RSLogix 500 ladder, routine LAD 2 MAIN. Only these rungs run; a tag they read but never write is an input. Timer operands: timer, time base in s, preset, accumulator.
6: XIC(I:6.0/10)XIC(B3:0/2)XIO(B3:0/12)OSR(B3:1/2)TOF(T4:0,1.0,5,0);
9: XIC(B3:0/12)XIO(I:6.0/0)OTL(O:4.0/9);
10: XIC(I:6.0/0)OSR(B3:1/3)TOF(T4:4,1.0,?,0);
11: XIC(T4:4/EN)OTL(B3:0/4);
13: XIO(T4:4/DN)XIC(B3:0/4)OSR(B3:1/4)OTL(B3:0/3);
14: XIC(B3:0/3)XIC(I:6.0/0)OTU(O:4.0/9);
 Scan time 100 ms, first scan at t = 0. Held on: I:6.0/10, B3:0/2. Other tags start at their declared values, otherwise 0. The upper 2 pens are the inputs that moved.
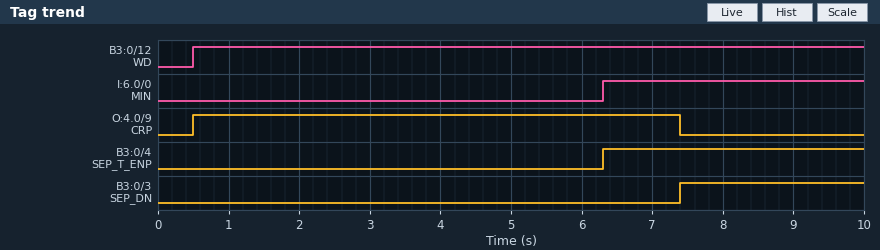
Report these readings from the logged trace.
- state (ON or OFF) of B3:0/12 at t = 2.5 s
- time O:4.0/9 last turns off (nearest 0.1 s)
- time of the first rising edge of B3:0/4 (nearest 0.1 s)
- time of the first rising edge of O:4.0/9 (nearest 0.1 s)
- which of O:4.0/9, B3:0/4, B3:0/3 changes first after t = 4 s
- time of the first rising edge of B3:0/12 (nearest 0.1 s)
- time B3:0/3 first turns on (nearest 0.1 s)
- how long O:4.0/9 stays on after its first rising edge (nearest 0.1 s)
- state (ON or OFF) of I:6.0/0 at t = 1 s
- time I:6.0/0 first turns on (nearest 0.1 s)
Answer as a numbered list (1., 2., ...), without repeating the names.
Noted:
1. ON
2. 7.4 s
3. 6.3 s
4. 0.5 s
5. B3:0/4
6. 0.5 s
7. 7.4 s
8. 6.9 s
9. OFF
10. 6.3 s
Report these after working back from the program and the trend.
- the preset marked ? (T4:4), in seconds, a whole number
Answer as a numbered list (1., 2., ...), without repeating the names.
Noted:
1. 1 s
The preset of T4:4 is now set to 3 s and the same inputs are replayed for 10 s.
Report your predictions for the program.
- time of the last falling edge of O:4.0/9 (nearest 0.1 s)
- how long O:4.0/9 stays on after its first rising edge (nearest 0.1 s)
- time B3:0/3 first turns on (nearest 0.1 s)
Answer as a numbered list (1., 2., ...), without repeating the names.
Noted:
1. 9.4 s
2. 8.9 s
3. 9.4 s
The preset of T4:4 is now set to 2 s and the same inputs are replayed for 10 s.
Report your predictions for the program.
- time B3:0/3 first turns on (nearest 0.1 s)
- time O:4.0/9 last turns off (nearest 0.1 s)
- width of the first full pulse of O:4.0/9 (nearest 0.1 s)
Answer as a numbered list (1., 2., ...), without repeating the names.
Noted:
1. 8.4 s
2. 8.4 s
3. 7.9 s
